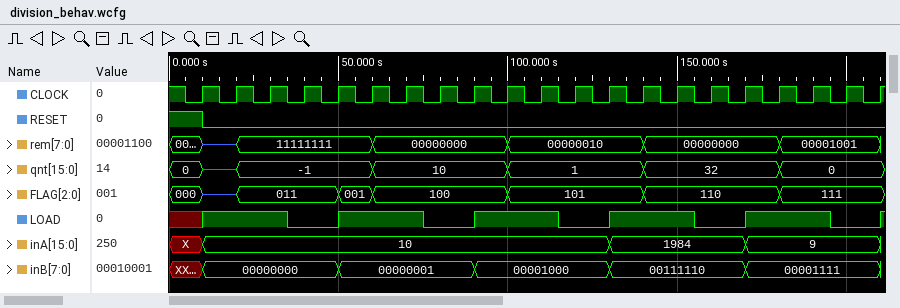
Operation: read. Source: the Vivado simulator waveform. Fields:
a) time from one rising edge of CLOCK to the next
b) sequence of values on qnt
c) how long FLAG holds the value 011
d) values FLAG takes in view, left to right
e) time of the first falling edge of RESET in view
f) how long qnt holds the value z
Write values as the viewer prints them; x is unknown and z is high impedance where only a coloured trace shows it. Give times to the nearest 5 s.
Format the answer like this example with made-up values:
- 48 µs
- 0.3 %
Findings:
- 10 s
- 0, z, -1, 10, 1, 32, 0
- 30 s
- 000, z, 011, 001, 100, 101, 110, 111
- 10 s
- 10 s
